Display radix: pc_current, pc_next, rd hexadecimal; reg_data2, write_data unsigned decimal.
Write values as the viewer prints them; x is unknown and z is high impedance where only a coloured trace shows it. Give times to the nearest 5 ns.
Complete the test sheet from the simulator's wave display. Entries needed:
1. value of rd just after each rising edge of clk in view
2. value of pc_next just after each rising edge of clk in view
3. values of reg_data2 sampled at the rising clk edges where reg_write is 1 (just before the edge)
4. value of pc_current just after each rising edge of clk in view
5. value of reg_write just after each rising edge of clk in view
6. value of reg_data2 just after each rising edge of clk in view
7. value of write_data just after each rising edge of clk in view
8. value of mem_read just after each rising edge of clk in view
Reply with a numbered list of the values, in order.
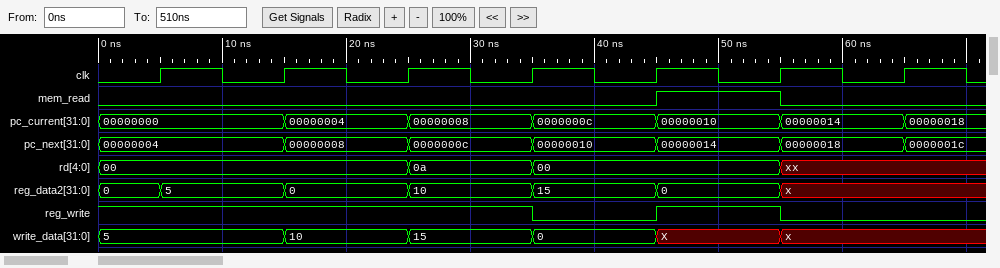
1. 00, 00, 0a, 00, 00, xx, xx
2. 00000004, 00000008, 0000000c, 00000010, 00000014, 00000018, 0000001c
3. 0, 5, 0, 10, 0
4. 00000000, 00000004, 00000008, 0000000c, 00000010, 00000014, 00000018
5. 1 1 1 0 1 0 0
6. 5, 0, 10, 15, 0, x, x
7. 5, 10, 15, 0, X, x, x
8. 0 0 0 0 1 0 0
